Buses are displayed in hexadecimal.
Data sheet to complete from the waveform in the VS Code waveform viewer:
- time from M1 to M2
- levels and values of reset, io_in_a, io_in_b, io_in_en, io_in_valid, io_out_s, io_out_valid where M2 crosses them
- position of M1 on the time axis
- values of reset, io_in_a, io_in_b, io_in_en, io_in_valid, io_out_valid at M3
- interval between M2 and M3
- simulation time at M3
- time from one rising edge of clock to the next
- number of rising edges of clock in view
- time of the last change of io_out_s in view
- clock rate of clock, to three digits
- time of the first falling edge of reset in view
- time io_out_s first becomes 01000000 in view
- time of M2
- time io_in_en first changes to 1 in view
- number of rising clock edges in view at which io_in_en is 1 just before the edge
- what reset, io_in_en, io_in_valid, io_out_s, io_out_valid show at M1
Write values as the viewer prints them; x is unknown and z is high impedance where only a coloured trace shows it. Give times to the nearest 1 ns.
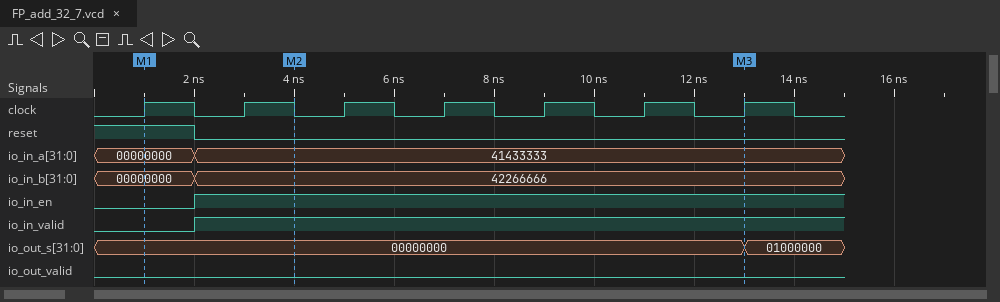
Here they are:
3 ns
reset=0, io_in_a=41433333, io_in_b=42266666, io_in_en=1, io_in_valid=1, io_out_s=00000000, io_out_valid=0
1 ns
reset=0, io_in_a=41433333, io_in_b=42266666, io_in_en=1, io_in_valid=1, io_out_valid=0
9 ns
13 ns
2 ns
7
13 ns
500 MHz
2 ns
13 ns
4 ns
2 ns
6
reset=1, io_in_en=0, io_in_valid=0, io_out_s=00000000, io_out_valid=0
